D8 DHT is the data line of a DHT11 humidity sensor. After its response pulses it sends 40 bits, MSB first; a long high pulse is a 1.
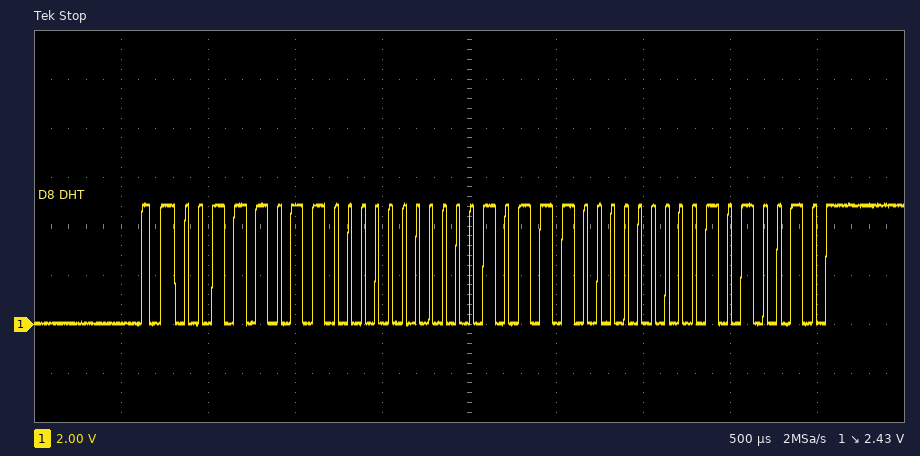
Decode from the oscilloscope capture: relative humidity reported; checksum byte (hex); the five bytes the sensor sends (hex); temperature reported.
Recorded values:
59 %
0x52
3B 00 17 00 52
23.0 °C
